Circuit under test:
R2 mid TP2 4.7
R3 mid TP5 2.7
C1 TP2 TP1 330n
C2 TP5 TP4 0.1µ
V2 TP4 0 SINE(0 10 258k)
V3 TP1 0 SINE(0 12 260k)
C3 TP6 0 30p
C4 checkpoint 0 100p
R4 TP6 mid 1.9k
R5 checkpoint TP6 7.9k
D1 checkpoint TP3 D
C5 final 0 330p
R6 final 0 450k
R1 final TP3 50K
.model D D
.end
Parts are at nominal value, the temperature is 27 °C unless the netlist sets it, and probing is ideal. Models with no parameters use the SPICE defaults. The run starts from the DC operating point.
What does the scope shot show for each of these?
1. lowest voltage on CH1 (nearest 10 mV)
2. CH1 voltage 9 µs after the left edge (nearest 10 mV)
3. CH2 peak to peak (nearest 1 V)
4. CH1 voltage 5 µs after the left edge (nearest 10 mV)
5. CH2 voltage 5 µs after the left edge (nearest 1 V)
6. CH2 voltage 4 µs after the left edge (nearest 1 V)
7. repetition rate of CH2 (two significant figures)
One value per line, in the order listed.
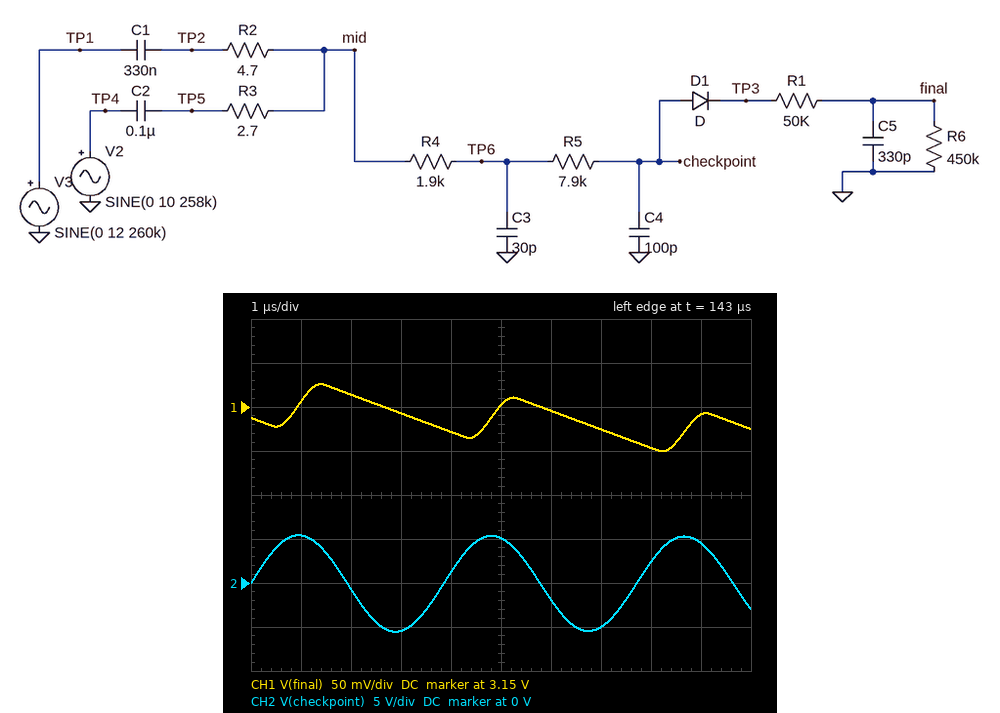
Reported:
3.10 V
3.14 V
11 V
3.15 V
5 V
1 V
260 kHz
